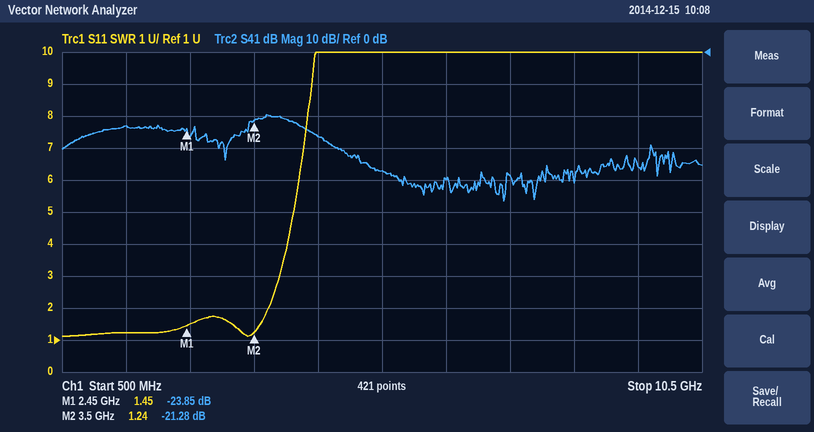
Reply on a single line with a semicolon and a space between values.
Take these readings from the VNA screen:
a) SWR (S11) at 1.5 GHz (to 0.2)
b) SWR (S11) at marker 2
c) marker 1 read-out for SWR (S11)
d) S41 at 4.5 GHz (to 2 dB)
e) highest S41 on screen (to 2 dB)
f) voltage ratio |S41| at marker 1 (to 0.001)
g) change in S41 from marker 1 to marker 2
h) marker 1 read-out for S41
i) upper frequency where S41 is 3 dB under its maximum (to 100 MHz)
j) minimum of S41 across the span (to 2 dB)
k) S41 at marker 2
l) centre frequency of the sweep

1.2; 1.24; 1.45; -26 dB; -20 dB; 0.064; 2.57 dB; -23.85 dB; 4.2 GHz; -46 dB; -21.28 dB; 5.5 GHz
